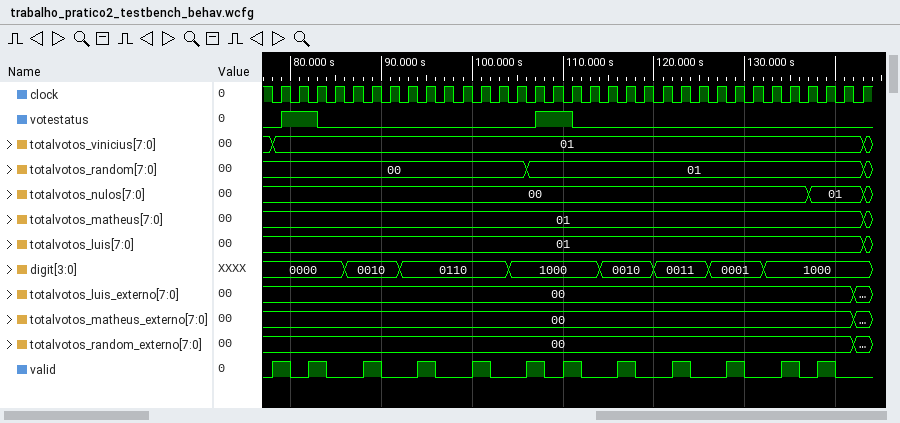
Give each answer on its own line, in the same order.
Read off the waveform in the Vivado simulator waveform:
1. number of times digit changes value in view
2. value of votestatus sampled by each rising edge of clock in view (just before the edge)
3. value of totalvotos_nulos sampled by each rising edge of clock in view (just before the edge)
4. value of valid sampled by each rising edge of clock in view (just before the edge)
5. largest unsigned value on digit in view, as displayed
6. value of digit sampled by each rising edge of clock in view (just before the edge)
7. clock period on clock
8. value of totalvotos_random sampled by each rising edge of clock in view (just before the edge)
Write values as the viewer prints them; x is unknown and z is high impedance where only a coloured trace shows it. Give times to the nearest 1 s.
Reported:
7
0 1 1 0 0 0 0 0 0 0 0 0 0 0 0 1 1 0 0 0 0 0 0 0 0 0 0 0 0 0 0 0 0
00, 00, 00, 00, 00, 00, 00, 00, 00, 00, 00, 00, 00, 00, 00, 00, 00, 00, 00, 00, 00, 00, 00, 00, 00, 00, 00, 00, 00, 00, 01, 01, 01
1 0 1 0 0 1 0 0 1 0 0 1 0 0 1 0 1 0 0 1 0 0 1 0 0 1 0 0 1 0 1 0 0
1000
0000, 0000, 0000, 0000, 0010, 0010, 0010, 0110, 0110, 0110, 0110, 0110, 0110, 1000, 1000, 1000, 1000, 1000, 0010, 0010, 0010, 0011, 0011, 0011, 0001, 0001, 0001, 1000, 1000, 1000, 1000, 1000, 1000
2 s
00, 00, 00, 00, 00, 00, 00, 00, 00, 00, 00, 00, 00, 00, 01, 01, 01, 01, 01, 01, 01, 01, 01, 01, 01, 01, 01, 01, 01, 01, 01, 01, 01
